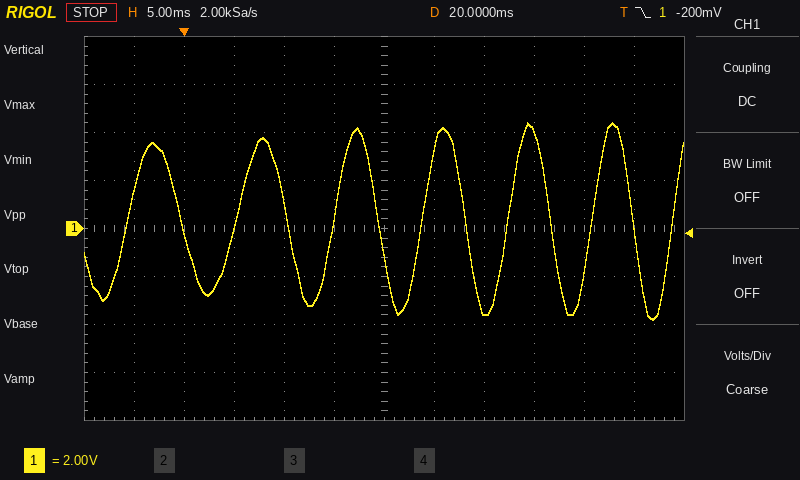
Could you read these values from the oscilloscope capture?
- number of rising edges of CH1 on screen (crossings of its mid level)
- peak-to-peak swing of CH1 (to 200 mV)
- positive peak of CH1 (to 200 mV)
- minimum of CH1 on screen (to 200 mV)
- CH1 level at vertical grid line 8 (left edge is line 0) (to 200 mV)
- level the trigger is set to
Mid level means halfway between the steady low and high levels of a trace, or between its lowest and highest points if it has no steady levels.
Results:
7
8.2 V
4.4 V
-3.8 V
-3.4 V
-200 mV
